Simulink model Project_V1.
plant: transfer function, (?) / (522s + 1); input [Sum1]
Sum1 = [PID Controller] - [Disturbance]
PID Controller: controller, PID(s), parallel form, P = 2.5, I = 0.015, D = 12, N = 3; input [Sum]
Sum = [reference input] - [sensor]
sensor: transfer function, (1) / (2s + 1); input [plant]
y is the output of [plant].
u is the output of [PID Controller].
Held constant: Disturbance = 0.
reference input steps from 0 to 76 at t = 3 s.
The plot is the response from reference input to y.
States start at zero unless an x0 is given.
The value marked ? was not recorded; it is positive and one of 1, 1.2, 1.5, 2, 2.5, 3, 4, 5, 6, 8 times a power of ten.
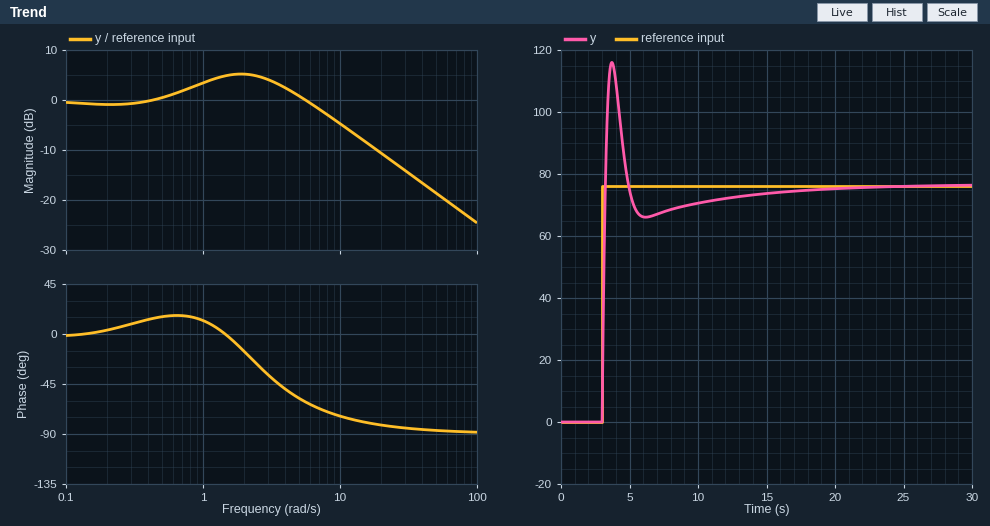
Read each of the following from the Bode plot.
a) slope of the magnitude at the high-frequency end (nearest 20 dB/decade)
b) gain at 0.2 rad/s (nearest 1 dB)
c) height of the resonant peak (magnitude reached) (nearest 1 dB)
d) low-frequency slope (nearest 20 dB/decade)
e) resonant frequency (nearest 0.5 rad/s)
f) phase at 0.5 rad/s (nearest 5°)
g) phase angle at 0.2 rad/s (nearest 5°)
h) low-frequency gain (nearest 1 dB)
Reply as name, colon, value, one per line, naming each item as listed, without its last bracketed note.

slope of the magnitude at the high-frequency end: -20 dB/decade
gain at 0.2 rad/s: -1 dB
height of the resonant peak (magnitude reached): 5 dB
low-frequency slope: 0 dB/decade
resonant frequency: 2.0 rad/s
phase at 0.5 rad/s: 15°
phase angle at 0.2 rad/s: 5°
low-frequency gain: -1 dB
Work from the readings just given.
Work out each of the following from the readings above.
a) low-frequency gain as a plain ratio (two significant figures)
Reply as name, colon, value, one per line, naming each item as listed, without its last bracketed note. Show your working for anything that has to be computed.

low-frequency gain as a plain ratio: 10^(-1 / 20) = 0.89
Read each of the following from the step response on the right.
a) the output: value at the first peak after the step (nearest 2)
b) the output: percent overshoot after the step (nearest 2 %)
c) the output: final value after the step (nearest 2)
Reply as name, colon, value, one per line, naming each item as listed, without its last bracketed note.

the output: value at the first peak after the step: 116
the output: percent overshoot after the step: 52 %
the output: final value after the step: 76
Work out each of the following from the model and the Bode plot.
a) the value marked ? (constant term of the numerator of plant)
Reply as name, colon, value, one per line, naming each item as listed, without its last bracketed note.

the value marked ?: 80
